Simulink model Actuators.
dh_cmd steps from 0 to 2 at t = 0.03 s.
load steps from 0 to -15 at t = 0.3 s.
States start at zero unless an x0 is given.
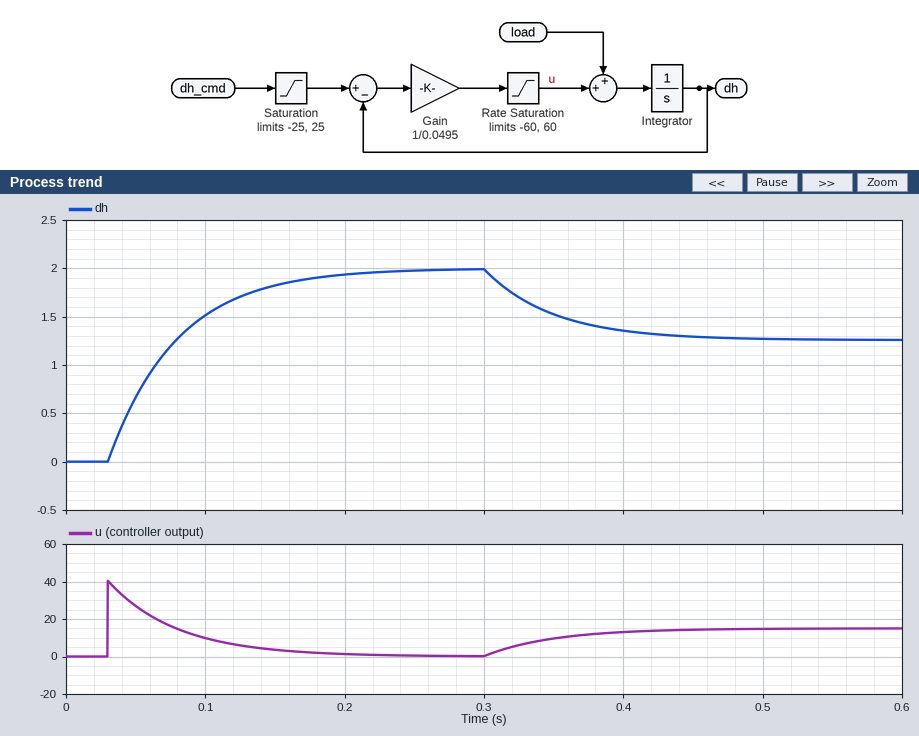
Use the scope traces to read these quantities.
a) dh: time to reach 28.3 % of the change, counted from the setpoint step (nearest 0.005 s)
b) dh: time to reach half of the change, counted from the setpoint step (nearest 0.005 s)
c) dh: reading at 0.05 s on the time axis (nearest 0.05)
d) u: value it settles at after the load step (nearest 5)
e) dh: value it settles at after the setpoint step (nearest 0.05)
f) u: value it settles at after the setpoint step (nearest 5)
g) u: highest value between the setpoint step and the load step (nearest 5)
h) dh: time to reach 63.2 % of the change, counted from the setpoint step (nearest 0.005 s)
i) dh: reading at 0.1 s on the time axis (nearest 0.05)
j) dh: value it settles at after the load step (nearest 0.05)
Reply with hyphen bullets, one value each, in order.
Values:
- 0.015 s
- 0.035 s
- 0.65
- 15
- 2.00
- 0
- 40
- 0.050 s
- 1.50
- 1.25
